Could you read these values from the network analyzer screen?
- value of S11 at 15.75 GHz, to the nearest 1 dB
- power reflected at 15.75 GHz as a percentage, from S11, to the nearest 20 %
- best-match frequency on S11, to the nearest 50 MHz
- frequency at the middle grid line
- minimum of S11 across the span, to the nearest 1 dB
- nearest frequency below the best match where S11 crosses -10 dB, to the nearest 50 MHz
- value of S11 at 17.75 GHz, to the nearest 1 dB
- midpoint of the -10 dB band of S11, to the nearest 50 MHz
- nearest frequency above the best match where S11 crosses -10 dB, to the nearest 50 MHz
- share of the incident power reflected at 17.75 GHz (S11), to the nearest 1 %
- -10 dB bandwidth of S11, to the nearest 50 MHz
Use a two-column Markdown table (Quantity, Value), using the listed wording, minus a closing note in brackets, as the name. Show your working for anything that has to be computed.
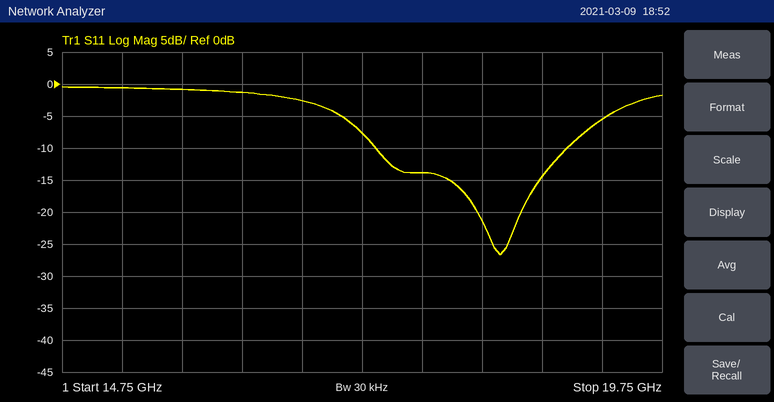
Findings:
| Quantity | Value |
|---|---|
| value of S11 at 15.75 GHz, to the nearest 1 dB | -1 dB |
| power reflected at 15.75 GHz as a percentage, from S11, to the nearest 20 % | 10^(-1/10) ≈ 79.4 %, so 80 % to the nearest 20 % |
| best-match frequency on S11, to the nearest 50 MHz | 18.40 GHz |
| frequency at the middle grid line | 17.25 GHz |
| minimum of S11 across the span, to the nearest 1 dB | -27 dB |
| nearest frequency below the best match where S11 crosses -10 dB, to the nearest 50 MHz | 17.35 GHz |
| value of S11 at 17.75 GHz, to the nearest 1 dB | -14 dB |
| midpoint of the -10 dB band of S11, to the nearest 50 MHz | 18.15 GHz |
| nearest frequency above the best match where S11 crosses -10 dB, to the nearest 50 MHz | 18.95 GHz |
| share of the incident power reflected at 17.75 GHz (S11), to the nearest 1 % | 10^(-14/10) ≈ 4 % |
| -10 dB bandwidth of S11, to the nearest 50 MHz | 18.95 GHz − 17.35 GHz = 1.60 GHz |
